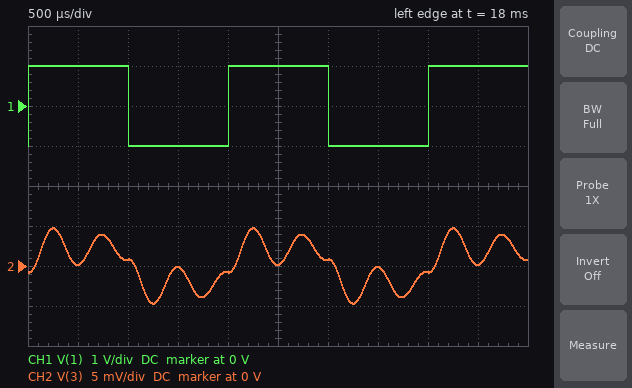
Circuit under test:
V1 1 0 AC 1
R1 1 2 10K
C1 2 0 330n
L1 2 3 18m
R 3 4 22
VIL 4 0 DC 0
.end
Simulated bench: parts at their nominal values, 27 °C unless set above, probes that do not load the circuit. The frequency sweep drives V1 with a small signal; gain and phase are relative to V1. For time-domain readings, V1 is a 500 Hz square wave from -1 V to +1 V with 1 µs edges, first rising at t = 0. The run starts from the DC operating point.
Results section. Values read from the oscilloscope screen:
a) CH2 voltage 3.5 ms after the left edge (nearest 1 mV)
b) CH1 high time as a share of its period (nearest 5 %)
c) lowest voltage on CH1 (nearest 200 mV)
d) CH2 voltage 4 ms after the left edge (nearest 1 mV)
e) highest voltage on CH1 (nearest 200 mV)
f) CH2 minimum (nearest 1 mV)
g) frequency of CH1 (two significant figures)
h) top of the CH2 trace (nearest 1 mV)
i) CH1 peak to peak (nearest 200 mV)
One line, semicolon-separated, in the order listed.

0 V; 50 %; -1.0 V; -1 mV; 1.0 V; -5 mV; 500 Hz; 5 mV; 2.0 V
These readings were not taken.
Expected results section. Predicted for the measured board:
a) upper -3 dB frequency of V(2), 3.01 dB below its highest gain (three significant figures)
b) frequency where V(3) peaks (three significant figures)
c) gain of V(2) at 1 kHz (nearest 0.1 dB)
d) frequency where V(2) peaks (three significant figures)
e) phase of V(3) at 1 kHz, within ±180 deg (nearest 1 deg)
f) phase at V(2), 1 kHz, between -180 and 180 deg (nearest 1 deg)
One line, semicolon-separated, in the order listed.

2.19 kHz; 2.06 kHz; -36.5 dB; 2.07 kHz; -4 deg; 75 deg
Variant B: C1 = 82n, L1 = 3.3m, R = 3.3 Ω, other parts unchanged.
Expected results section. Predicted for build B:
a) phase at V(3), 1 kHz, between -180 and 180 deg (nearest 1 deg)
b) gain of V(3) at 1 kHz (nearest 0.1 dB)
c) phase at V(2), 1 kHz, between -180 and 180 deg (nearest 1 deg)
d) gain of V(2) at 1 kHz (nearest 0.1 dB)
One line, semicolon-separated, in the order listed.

0 deg; -69.5 dB; 81 deg; -53.5 dB
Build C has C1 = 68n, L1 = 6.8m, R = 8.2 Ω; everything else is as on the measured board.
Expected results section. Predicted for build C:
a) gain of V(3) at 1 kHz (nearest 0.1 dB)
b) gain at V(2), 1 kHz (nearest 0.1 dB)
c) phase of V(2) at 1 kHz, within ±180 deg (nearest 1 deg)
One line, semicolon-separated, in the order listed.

-61.6 dB; -47.1 dB; 79 deg
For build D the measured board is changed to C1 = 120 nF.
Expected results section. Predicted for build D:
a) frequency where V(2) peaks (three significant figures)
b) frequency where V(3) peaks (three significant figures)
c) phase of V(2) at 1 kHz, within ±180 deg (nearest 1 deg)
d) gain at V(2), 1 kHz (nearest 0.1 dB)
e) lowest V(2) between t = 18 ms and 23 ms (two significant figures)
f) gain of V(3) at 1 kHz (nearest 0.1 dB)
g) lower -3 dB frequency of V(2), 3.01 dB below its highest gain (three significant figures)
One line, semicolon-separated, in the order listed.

3.43 kHz; 3.42 kHz; 77 deg; -38.0 dB; -100 mV; -52.4 dB; 3.27 kHz
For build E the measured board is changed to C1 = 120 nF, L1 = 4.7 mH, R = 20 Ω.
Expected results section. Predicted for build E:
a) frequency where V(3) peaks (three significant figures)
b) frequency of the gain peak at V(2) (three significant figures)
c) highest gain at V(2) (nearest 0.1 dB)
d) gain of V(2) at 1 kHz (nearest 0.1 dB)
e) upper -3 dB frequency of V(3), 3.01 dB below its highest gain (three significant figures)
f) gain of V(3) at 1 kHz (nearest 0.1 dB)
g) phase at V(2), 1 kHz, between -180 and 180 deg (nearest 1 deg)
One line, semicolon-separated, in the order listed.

6.68 kHz; 6.71 kHz; -15.7 dB; -48.8 dB; 7.08 kHz; -53.8 dB; 55 deg
